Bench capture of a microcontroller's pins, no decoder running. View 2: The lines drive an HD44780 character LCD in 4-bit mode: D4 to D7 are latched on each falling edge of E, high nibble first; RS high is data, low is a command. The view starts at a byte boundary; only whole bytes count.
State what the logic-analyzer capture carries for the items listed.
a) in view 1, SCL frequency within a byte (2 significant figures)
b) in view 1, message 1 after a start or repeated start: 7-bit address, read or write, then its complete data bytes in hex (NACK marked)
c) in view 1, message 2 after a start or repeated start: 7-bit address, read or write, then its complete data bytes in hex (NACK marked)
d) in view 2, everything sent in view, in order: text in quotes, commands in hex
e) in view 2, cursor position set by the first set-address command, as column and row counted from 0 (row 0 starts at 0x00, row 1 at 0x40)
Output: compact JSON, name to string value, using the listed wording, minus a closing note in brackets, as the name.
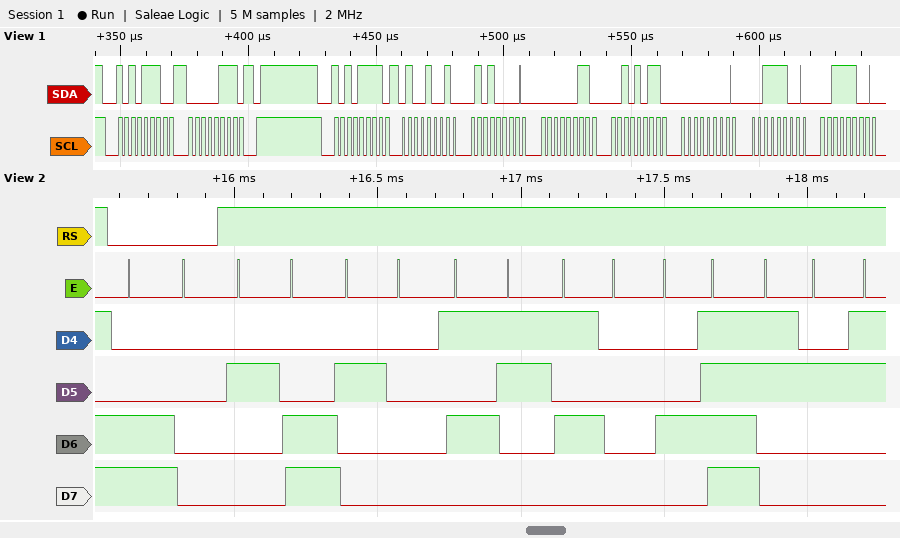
{"in view 1, SCL frequency within a byte": "400 kHz", "in view 1, message 1 after a start or repeated start: 7-bit address, read or write, then its complete data bytes in hex": "0x57 write: 07", "in view 1, message 2 after a start or repeated start: 7-bit address, read or write, then its complete data bytes in hex": "0x57 read: 49 50 03 2B 00 3C 3C", "in view 2, everything sent in view, in order: text in quotes, commands in hex": "0xC0 \", SPO2\"", "in view 2, cursor position set by the first set-address command, as column and row counted from 0": "column 0, row 1"}
